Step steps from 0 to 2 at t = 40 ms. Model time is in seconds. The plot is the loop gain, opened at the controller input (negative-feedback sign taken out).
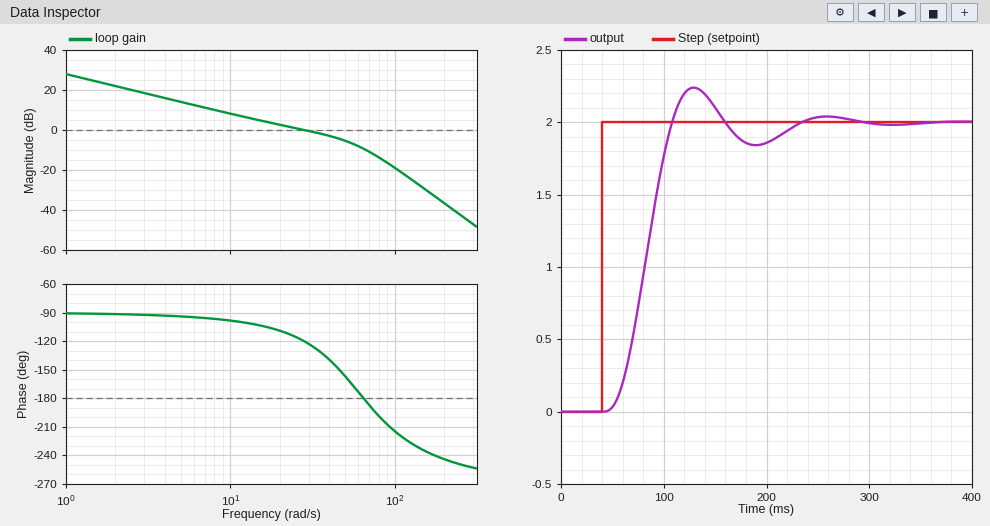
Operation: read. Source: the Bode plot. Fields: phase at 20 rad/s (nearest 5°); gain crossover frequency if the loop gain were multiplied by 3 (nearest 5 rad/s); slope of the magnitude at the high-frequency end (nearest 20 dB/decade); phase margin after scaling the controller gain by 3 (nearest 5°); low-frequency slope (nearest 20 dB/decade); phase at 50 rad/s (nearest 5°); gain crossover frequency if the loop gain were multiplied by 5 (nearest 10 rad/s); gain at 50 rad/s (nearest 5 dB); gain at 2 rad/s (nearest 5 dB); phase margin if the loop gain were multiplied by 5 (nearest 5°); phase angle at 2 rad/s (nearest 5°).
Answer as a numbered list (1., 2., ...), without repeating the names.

1. -110°
2. 65 rad/s
3. -60 dB/decade
4. 0°
5. -20 dB/decade
6. -155°
7. 80 rad/s
8. -5 dB
9. 20 dB
10. -20°
11. -90°
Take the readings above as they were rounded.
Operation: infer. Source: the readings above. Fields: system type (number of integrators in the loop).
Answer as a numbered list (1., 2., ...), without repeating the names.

1. 1
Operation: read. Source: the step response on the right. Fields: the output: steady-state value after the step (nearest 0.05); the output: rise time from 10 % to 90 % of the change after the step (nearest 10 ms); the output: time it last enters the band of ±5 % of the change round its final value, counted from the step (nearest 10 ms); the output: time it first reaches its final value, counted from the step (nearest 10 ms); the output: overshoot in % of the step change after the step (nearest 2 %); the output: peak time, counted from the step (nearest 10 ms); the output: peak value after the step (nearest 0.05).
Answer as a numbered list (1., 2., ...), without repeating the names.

1. 2.00
2. 40 ms
3. 170 ms
4. 70 ms
5. 12 %
6. 90 ms
7. 2.25
